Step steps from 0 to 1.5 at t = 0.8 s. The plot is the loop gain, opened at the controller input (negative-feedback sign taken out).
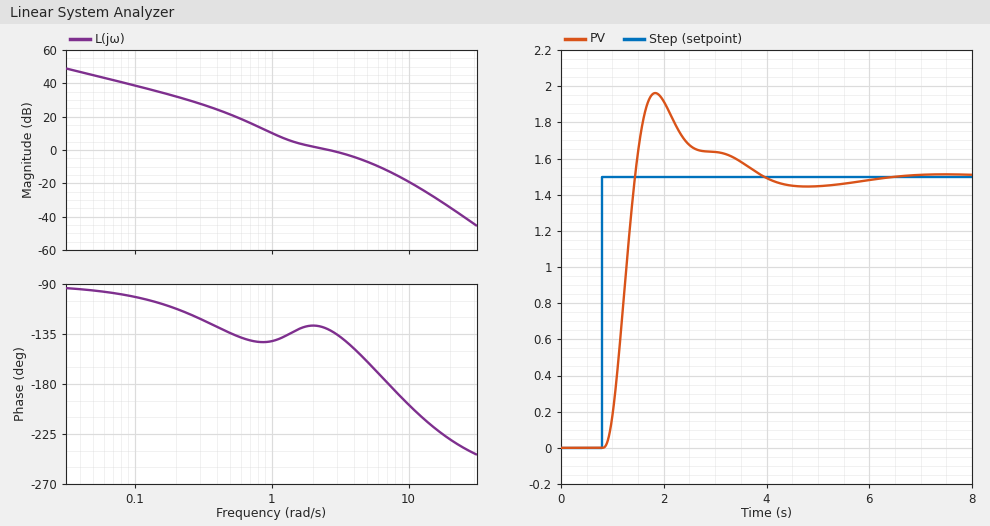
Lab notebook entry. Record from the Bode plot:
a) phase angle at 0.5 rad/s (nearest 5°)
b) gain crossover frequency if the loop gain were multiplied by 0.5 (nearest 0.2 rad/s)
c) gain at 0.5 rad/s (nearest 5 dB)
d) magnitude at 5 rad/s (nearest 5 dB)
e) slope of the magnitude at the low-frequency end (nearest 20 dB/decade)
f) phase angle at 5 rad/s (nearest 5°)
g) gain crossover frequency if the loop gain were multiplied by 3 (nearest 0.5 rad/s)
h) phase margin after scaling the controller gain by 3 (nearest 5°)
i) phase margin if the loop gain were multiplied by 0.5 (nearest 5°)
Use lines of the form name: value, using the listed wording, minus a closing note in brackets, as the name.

phase angle at 0.5 rad/s: -135°
gain crossover frequency if the loop gain were multiplied by 0.5: 1.4 rad/s
gain at 0.5 rad/s: 20 dB
magnitude at 5 rad/s: -5 dB
slope of the magnitude at the low-frequency end: -20 dB/decade
phase angle at 5 rad/s: -160°
gain crossover frequency if the loop gain were multiplied by 3: 6.0 rad/s
phase margin after scaling the controller gain by 3: 10°
phase margin if the loop gain were multiplied by 0.5: 45°
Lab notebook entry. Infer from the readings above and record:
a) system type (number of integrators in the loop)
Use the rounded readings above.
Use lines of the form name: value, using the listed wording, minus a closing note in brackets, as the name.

system type: 1
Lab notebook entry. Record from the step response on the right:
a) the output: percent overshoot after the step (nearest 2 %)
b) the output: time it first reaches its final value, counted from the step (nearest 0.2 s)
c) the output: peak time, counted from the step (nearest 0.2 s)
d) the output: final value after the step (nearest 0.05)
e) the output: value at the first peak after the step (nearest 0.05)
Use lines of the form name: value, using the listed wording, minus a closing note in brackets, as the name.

the output: percent overshoot after the step: 30 %
the output: time it first reaches its final value, counted from the step: 0.6 s
the output: peak time, counted from the step: 1.0 s
the output: final value after the step: 1.50
the output: value at the first peak after the step: 1.95
